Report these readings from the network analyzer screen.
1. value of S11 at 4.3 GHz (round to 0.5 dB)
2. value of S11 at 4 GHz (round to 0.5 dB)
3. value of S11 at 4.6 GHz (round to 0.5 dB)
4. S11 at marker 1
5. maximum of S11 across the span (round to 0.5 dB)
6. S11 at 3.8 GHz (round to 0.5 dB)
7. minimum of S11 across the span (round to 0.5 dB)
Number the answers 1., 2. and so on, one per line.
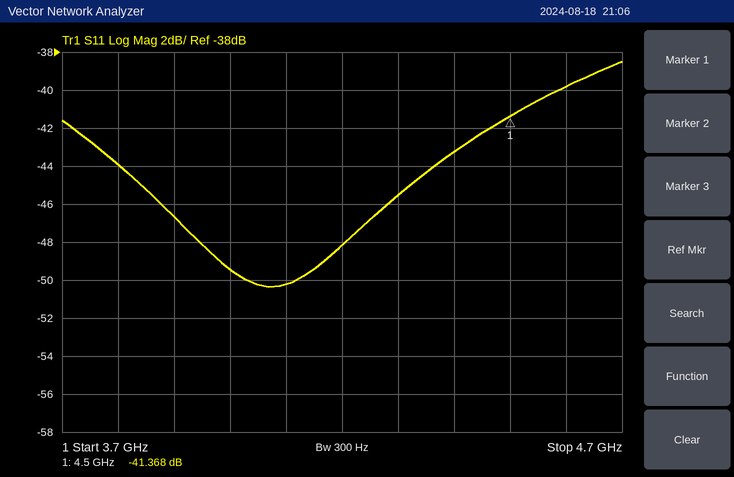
1. -45.5 dB
2. -49.5 dB
3. -40.0 dB
4. -41.368 dB
5. -38.5 dB
6. -44.0 dB
7. -50.5 dB
